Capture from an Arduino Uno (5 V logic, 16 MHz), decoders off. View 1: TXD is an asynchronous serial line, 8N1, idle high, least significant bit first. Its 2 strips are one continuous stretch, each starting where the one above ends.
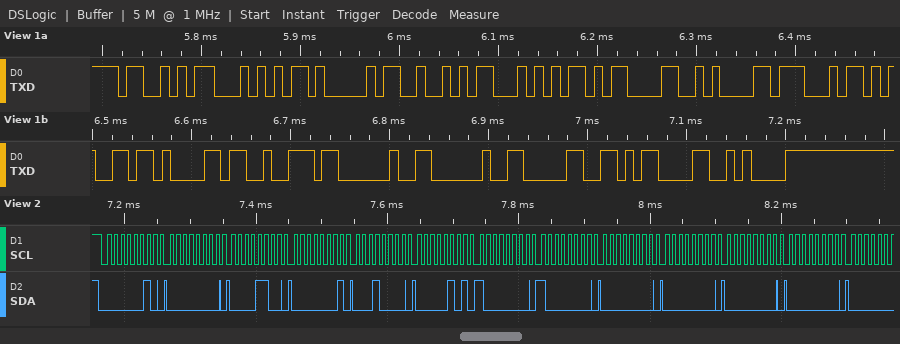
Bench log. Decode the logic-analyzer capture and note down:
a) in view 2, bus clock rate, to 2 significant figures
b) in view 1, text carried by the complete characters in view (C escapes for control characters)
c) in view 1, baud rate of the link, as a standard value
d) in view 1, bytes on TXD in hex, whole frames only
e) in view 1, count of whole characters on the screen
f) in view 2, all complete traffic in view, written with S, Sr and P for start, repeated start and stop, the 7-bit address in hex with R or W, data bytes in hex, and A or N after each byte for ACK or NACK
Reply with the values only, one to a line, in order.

100 kHz
"START\r\nGear  0\r\n"
115200 baud
0x53 0x54 0x41 0x52 0x54 0x0D 0x0A 0x47 0x65 0x61 0x72 0x20 0x20 0x30 0x0D 0x0A
16
S 01W A 00 A 0C A 01 A 10 A 05 A 80 A 80 A 00 A 00 A 00 A 00 A
